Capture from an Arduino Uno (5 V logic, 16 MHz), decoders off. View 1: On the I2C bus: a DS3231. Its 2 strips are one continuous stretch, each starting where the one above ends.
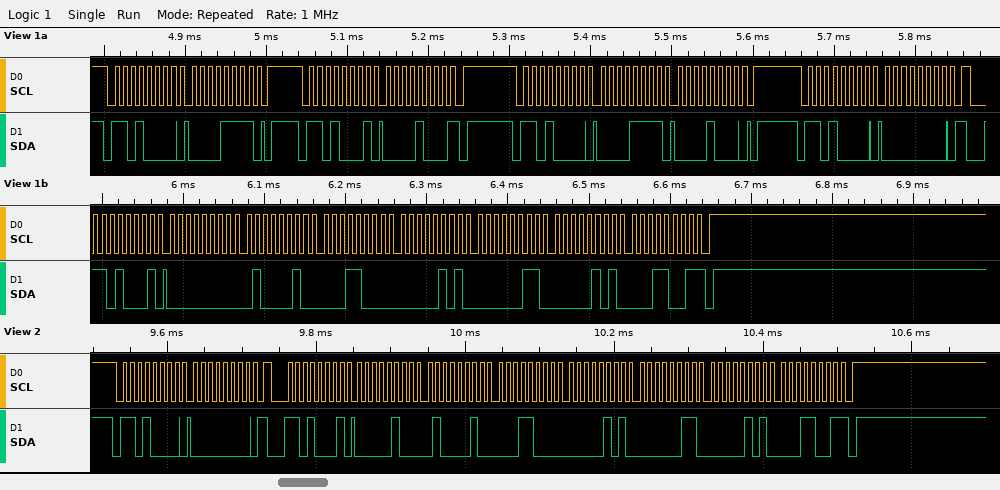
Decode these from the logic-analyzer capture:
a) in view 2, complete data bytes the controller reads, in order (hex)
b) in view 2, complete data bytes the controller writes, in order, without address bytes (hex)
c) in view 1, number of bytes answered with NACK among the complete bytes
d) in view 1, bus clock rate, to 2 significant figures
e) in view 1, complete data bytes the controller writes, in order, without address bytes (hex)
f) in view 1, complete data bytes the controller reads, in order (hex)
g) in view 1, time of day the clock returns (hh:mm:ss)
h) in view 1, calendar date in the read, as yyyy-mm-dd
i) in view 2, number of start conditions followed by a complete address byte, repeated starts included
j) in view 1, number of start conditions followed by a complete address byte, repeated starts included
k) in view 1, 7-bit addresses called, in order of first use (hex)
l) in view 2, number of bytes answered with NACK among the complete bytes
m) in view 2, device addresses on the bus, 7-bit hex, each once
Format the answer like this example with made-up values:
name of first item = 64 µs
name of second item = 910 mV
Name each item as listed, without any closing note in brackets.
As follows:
in view 2, complete data bytes the controller reads, in order = 04 42 18 05 03 05 19
in view 2, complete data bytes the controller writes, in order, without address bytes = 00
in view 1, number of bytes answered with NACK among the complete bytes = 2
in view 1, bus clock rate, to 2 significant figures = 100 kHz
in view 1, complete data bytes the controller writes, in order, without address bytes = 0F 0F 08 00
in view 1, complete data bytes the controller reads, in order = 08 00 42 18 05 03 05 19
in view 1, time of day the clock returns = 18:42:00
in view 1, calendar date in the read, as yyyy-mm-dd = 2019-05-03
in view 2, number of start conditions followed by a complete address byte, repeated starts included = 2
in view 1, number of start conditions followed by a complete address byte, repeated starts included = 5
in view 1, 7-bit addresses called, in order of first use = 0x68
in view 2, number of bytes answered with NACK among the complete bytes = 1
in view 2, device addresses on the bus, 7-bit hex, each once = 0x68
